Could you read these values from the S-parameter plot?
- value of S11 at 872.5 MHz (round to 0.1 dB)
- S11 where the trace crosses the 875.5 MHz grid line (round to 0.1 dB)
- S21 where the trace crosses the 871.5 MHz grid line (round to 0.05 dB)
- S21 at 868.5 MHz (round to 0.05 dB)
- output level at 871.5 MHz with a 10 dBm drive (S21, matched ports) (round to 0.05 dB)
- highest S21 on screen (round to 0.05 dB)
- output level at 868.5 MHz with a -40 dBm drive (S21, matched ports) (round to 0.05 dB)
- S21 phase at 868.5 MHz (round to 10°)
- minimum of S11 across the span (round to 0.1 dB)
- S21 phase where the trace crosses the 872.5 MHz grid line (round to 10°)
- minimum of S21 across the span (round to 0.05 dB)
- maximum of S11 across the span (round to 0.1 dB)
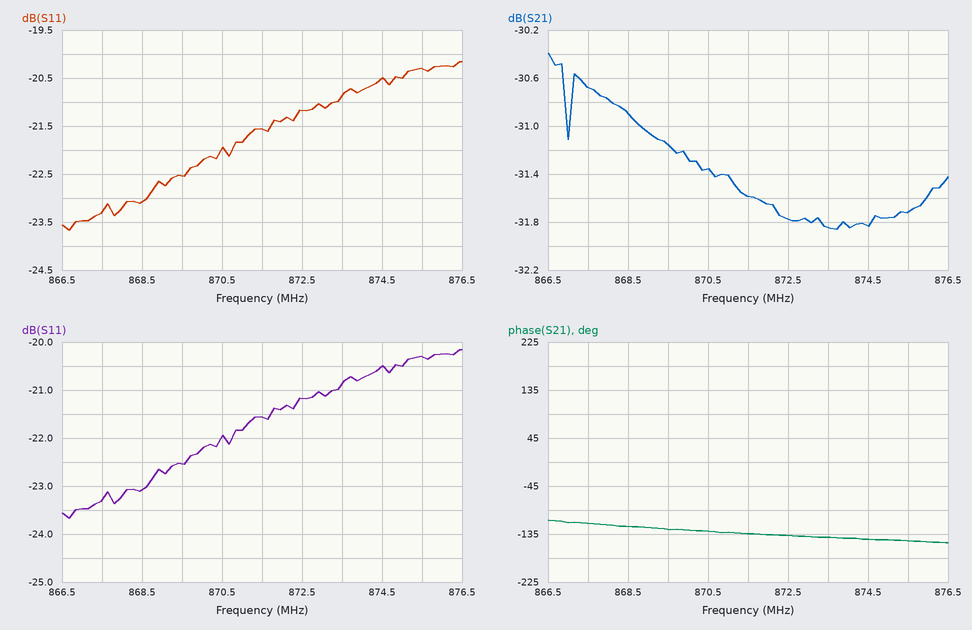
-21.2 dB
-20.3 dB
-31.60 dB
-30.90 dB
-21.60 dBm
-30.40 dB
-70.90 dBm
-120°
-23.7 dB
-140°
-31.85 dB
-20.2 dB
